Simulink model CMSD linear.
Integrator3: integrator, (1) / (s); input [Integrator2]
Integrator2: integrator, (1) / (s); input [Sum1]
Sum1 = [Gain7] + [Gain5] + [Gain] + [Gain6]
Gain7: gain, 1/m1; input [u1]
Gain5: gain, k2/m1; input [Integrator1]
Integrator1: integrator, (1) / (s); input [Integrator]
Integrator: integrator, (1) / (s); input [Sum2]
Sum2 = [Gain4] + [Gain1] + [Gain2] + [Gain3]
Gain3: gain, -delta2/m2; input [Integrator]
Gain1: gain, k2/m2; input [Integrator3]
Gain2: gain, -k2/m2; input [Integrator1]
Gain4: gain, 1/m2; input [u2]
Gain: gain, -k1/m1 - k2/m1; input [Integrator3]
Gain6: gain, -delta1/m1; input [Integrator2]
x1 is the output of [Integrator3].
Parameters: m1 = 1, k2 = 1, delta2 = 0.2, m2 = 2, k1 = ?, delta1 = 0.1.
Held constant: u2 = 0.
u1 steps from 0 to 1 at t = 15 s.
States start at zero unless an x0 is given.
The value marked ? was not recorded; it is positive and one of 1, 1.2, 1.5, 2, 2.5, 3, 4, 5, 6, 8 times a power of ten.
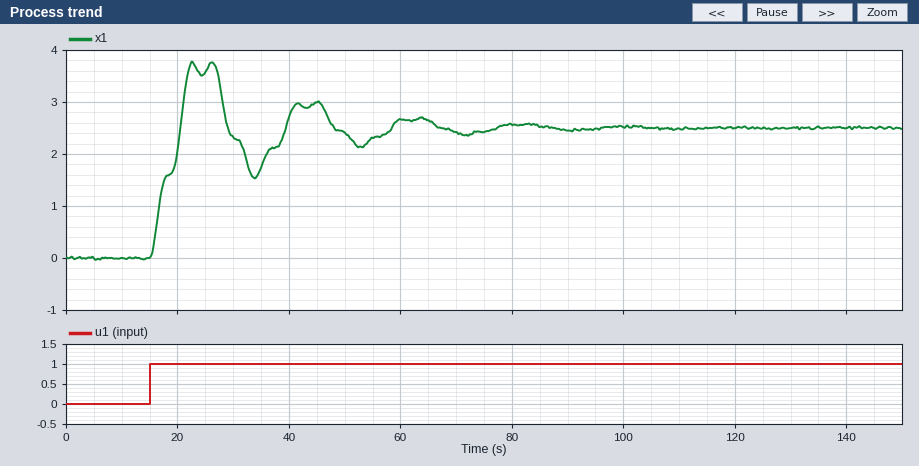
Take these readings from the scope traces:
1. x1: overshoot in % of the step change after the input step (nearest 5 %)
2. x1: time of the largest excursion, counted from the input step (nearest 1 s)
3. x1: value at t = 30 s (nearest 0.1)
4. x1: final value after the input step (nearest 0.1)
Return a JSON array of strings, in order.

["50 %", "11 s", "2.3", "2.5"]
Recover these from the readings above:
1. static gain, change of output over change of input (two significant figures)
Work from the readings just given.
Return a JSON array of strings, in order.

["2.5"]
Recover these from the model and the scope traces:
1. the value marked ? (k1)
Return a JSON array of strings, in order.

["0.4"]
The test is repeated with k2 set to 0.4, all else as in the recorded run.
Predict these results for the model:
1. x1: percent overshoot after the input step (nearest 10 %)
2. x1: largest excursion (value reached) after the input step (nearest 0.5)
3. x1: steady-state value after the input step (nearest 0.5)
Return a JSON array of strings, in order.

["60 %", "4.0", "2.5"]
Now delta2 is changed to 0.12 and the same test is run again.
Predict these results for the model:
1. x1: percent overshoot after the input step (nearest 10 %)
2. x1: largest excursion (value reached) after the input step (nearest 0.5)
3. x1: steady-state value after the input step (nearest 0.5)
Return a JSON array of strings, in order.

["60 %", "4.0", "2.5"]
